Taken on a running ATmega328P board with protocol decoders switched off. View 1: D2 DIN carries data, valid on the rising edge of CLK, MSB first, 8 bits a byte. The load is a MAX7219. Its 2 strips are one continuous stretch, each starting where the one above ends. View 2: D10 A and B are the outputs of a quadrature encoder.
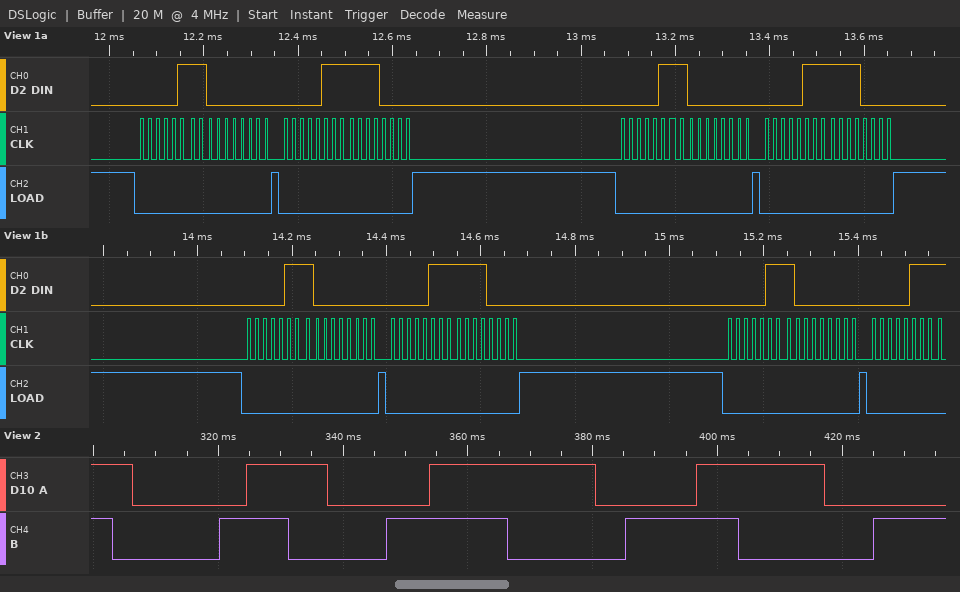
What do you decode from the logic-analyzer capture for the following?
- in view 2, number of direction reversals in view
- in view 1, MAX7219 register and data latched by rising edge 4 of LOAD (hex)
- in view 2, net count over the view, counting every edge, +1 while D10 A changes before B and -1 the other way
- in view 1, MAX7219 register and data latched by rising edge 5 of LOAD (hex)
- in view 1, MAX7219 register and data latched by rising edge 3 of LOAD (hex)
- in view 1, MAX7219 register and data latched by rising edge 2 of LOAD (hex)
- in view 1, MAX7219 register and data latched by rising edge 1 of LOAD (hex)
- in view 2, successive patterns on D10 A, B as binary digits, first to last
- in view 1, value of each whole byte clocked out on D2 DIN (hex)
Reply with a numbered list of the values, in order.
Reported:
1. 0
2. register 0x7, data 0xF0
3. -15
4. register 0x7, data 0x00
5. register 0x7, data 0x00
6. register 0x7, data 0xF0
7. register 0x7, data 0x00
8. 11 10 00 01 11 10 00 01 11 10 00 01 11 10 00 01
9. 0x07 0x00 0x07 0xF0 0x07 0x00 0x07 0xF0 0x07 0x00 0x07 0xF0 0x07 0x00 0x07
